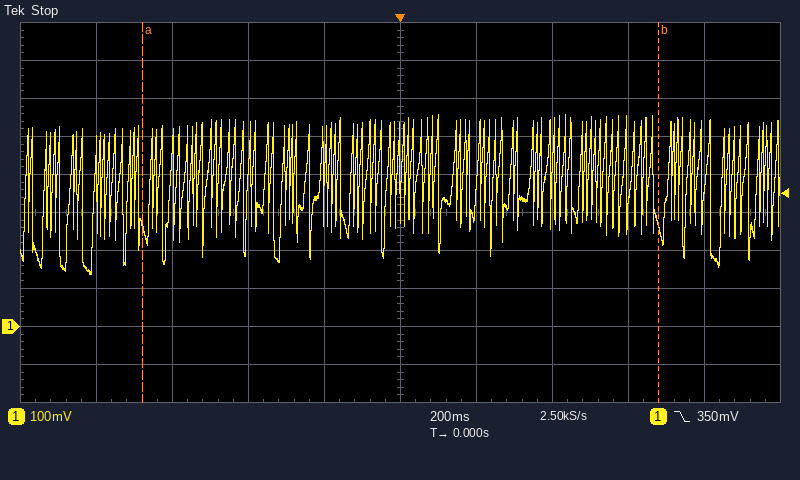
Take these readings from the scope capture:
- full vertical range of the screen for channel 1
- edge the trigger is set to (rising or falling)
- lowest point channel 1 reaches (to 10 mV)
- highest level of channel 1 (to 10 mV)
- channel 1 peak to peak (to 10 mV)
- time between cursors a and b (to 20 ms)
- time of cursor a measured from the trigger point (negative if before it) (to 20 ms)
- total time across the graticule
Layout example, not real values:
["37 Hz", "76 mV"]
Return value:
["1 V", "falling", "140 mV", "560 mV", "420 mV", "1.36 s", "-680 ms", "2 s"]
